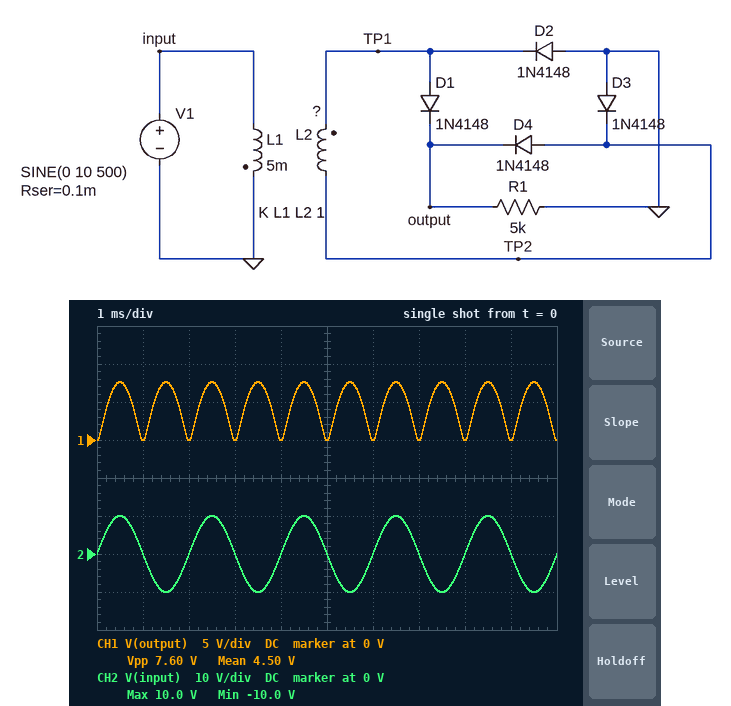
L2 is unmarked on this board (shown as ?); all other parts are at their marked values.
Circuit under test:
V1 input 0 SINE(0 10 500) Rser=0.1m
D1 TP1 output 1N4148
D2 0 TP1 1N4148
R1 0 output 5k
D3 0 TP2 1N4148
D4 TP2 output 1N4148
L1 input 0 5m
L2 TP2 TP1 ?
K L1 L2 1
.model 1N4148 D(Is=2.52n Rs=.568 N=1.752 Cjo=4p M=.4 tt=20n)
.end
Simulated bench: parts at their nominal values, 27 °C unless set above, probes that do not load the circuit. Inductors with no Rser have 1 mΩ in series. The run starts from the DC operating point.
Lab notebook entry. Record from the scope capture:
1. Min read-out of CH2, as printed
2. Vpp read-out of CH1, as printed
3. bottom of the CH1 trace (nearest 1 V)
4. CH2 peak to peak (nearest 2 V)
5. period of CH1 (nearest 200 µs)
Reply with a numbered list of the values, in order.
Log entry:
1. -10.0 V
2. 7.60 V
3. 0 V
4. 20 V
5. 1.0 ms
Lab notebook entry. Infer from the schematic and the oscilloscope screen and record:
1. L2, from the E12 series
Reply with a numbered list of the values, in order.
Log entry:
1. 3.9 mH
